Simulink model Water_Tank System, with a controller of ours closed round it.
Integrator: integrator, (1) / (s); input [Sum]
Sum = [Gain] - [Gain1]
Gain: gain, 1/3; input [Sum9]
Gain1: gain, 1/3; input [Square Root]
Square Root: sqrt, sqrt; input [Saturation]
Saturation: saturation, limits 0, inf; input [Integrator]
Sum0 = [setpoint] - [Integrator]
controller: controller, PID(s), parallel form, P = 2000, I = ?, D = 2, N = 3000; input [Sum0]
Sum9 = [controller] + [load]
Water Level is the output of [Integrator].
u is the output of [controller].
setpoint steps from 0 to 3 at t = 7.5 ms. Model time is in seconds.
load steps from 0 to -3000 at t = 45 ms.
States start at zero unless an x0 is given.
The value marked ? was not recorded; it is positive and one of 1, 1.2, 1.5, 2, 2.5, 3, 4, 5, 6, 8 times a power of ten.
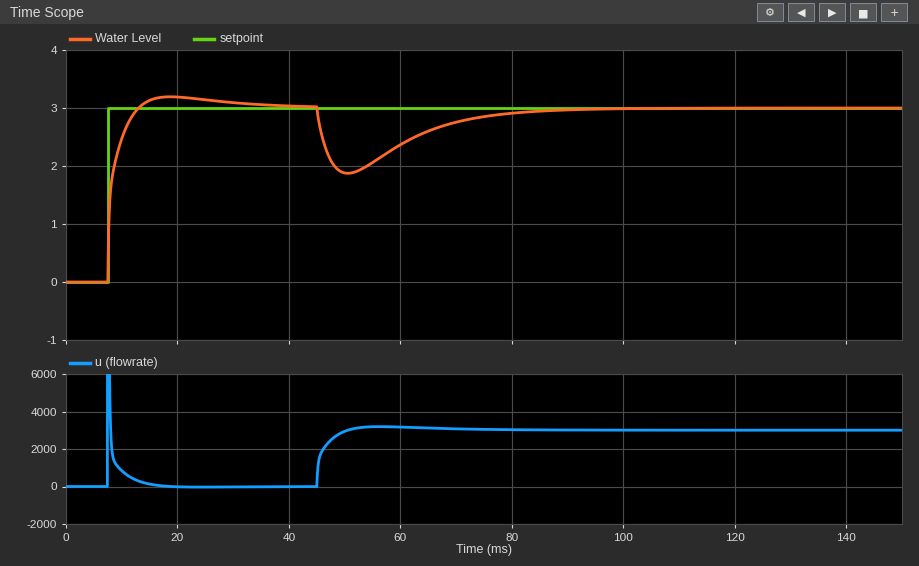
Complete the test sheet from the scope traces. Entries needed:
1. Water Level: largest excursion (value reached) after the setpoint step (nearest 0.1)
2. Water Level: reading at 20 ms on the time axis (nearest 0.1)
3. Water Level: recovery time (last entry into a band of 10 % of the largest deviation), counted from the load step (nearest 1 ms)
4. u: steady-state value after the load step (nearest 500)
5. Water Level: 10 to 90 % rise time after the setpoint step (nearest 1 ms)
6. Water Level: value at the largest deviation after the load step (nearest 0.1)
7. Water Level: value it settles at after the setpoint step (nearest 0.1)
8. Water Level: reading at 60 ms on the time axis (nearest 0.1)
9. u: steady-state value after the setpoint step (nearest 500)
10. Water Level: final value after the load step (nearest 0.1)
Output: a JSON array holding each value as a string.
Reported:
["3.2", "3.2", "33 ms", "3000", "3 ms", "1.9", "3.0", "2.4", "0", "3.0"]
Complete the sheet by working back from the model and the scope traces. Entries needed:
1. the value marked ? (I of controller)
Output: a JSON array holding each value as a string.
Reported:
["150000"]
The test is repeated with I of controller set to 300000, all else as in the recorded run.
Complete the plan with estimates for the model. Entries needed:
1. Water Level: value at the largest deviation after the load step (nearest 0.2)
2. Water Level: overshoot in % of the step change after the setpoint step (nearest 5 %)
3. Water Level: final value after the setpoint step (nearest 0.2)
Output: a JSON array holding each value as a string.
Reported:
["2.0", "10 %", "3.0"]
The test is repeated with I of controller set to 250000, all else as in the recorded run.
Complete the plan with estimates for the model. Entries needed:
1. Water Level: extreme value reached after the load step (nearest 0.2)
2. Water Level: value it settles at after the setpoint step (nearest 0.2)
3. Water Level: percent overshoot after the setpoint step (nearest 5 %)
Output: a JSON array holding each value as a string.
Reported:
["2.0", "3.0", "10 %"]
